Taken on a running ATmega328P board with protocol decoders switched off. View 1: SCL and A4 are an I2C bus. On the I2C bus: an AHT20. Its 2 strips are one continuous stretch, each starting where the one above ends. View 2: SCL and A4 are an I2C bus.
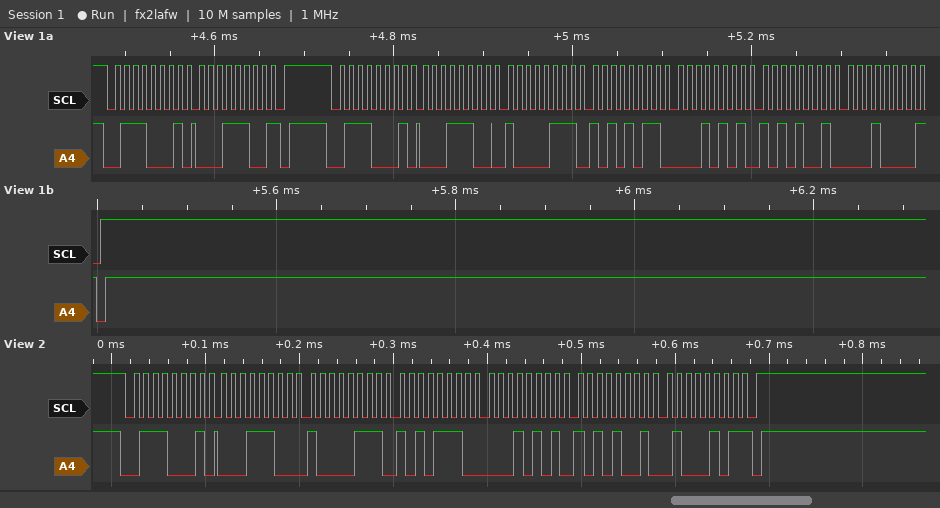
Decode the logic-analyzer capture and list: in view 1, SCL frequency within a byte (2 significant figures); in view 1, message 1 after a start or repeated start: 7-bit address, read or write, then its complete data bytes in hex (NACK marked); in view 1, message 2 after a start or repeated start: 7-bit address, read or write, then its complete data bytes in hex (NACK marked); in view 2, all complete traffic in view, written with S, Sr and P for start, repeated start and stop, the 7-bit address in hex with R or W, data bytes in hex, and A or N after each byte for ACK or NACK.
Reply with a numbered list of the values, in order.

1. 100 kHz
2. 0x38 read: 1C NACK
3. 0x38 read: 1C 87 AB 15 A9 10 NACK
4. S 38R A 1C A 87 A AE A 15 A A9 A 45 N P
